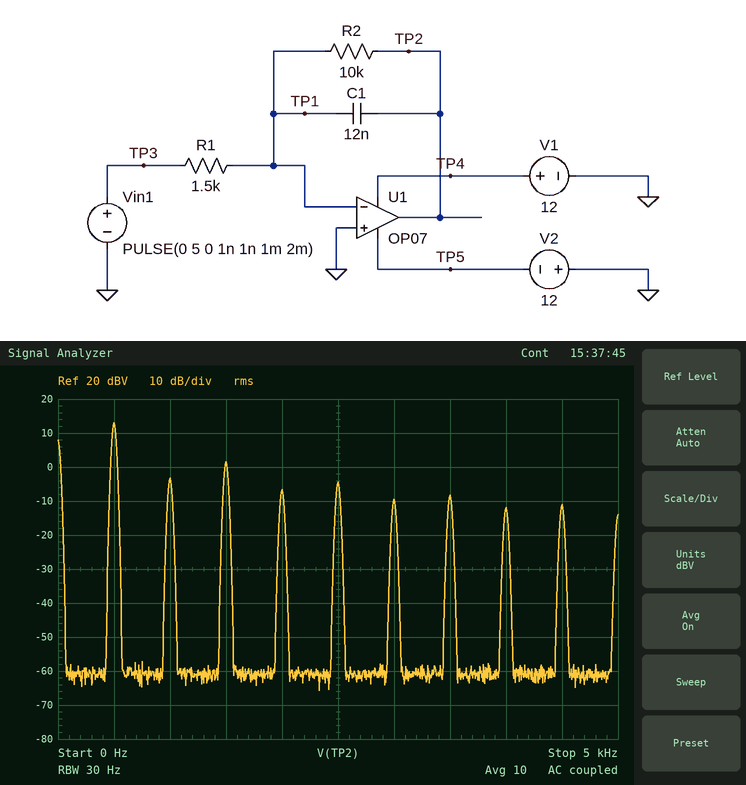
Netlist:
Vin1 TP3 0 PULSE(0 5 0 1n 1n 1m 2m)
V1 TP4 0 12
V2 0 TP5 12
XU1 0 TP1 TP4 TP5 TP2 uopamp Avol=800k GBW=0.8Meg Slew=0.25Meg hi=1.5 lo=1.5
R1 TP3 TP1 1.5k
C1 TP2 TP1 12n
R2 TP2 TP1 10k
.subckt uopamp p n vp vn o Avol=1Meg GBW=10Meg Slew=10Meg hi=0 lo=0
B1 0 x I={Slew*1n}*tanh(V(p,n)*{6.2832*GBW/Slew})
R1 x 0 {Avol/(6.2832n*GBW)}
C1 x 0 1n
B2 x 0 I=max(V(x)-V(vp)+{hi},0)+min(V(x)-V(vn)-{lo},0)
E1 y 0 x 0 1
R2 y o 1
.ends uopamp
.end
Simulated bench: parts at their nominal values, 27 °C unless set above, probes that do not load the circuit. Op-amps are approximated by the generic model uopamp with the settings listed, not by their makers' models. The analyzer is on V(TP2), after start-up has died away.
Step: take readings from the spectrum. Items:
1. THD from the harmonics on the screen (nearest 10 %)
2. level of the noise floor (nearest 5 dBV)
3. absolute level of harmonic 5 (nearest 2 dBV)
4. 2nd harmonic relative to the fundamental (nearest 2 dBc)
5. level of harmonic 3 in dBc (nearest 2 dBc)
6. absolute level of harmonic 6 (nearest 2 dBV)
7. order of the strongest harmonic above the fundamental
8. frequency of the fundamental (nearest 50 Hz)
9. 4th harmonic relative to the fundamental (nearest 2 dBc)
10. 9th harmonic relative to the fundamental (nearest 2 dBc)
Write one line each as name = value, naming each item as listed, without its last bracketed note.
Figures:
THD from the harmonics on the screen = 40 %
level of the noise floor = -60 dBV
absolute level of harmonic 5 = -4 dBV
2nd harmonic relative to the fundamental = -16 dBc
level of harmonic 3 in dBc = -12 dBc
absolute level of harmonic 6 = -10 dBV
order of the strongest harmonic above the fundamental = 3
frequency of the fundamental = 500 Hz
4th harmonic relative to the fundamental = -20 dBc
9th harmonic relative to the fundamental = -24 dBc
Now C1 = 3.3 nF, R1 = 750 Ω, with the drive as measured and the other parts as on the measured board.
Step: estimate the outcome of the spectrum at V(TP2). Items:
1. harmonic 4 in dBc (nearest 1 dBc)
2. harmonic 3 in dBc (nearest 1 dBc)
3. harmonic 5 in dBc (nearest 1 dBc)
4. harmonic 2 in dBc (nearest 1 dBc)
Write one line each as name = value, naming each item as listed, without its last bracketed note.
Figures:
harmonic 4 in dBc = -31 dBc
harmonic 3 in dBc = -10 dBc
harmonic 5 in dBc = -15 dBc
harmonic 2 in dBc = -30 dBc
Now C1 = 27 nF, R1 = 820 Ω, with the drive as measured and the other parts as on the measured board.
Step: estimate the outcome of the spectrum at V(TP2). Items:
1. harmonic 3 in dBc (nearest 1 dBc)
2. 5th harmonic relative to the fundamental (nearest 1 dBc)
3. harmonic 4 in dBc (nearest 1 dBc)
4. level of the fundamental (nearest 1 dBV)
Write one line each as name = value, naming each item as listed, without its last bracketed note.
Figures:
harmonic 3 in dBc = -13 dBc
5th harmonic relative to the fundamental = -18 dBc
harmonic 4 in dBc = -17 dBc
level of the fundamental = 12 dBV
